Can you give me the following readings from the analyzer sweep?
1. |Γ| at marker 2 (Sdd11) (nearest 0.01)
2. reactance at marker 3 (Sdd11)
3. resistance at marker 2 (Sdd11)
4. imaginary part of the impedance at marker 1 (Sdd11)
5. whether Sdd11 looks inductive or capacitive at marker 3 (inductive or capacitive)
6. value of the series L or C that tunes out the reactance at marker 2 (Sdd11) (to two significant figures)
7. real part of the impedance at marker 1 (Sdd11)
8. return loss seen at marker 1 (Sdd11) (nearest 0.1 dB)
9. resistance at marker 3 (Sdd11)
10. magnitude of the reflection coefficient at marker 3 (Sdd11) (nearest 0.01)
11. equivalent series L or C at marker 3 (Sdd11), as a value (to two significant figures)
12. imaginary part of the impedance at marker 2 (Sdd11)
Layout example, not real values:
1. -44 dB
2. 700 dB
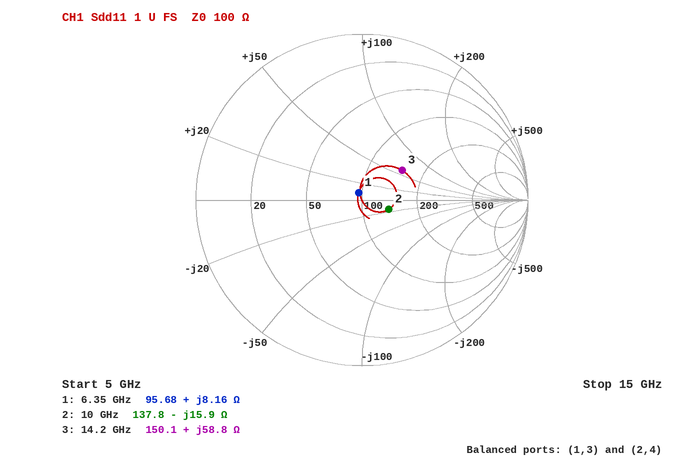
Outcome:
1. 0.17
2. +58.8 Ω
3. 137.8 Ω
4. +8.16 Ω
5. inductive
6. 250 pH
7. 95.68 Ω
8. 26.5 dB
9. 150.1 Ω
10. 0.30
11. 660 pH
12. -15.9 Ω
